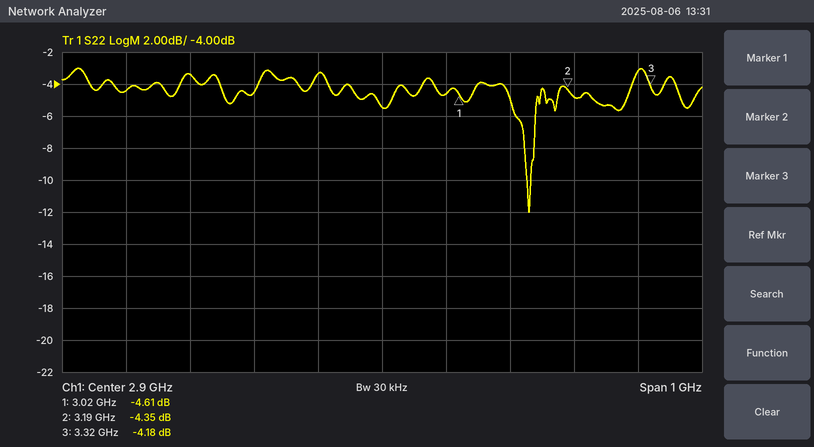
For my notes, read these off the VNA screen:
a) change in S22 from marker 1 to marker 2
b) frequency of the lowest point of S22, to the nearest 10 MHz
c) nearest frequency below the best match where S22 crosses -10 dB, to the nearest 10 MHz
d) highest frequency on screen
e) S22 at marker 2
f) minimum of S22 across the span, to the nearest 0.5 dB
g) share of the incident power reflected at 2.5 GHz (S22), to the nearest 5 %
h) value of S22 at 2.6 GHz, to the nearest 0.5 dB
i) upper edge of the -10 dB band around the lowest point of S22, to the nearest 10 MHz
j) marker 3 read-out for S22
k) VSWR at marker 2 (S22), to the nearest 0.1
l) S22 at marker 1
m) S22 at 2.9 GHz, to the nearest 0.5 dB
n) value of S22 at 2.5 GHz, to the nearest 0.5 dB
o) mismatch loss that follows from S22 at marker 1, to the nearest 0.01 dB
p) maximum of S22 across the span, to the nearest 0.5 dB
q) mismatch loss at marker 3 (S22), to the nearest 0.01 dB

0.26 dB
3.13 GHz
3.13 GHz
3.4 GHz
-4.35 dB
-12.0 dB
35 %
-3.5 dB
3.13 GHz
-4.18 dB
4.1
-4.61 dB
-5.5 dB
-4.5 dB
1.84 dB
-3.0 dB
2.09 dB
